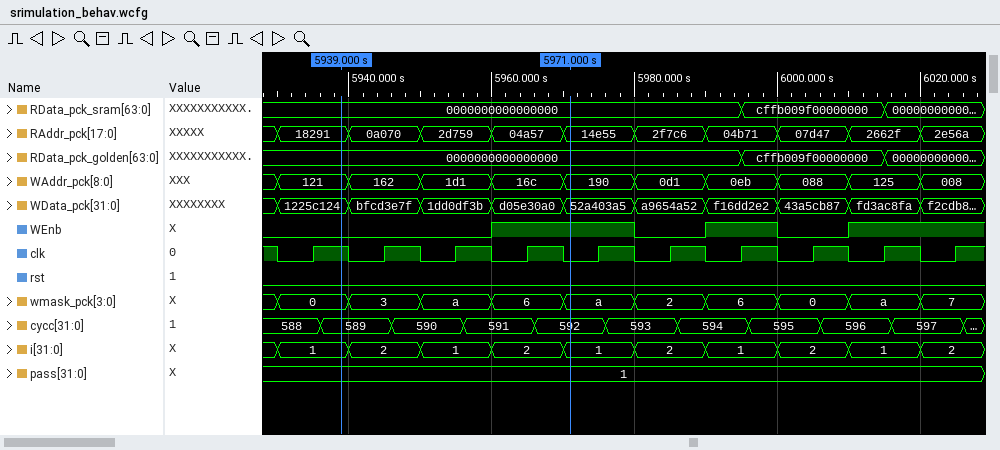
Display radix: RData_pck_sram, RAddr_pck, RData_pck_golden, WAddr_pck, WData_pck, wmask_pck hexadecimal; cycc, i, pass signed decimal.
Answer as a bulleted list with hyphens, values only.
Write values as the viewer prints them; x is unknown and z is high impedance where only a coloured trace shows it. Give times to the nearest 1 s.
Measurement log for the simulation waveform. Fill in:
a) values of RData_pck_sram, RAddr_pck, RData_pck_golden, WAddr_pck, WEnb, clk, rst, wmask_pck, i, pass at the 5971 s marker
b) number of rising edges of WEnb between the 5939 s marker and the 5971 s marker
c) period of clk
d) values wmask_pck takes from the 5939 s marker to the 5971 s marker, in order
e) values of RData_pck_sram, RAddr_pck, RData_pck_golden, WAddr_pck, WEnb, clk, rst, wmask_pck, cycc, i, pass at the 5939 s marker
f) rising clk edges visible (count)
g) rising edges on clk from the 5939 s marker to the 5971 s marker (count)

- RData_pck_sram=0000000000000000, RAddr_pck=14e55, RData_pck_golden=0000000000000000, WAddr_pck=190, WEnb=1, clk=0, rst=0, wmask_pck=a, i=1, pass=1
- 1
- 10 s
- 0, 3, a, 6, a
- RData_pck_sram=0000000000000000, RAddr_pck=18291, RData_pck_golden=0000000000000000, WAddr_pck=121, WEnb=0, clk=1, rst=0, wmask_pck=0, cycc=589, i=1, pass=1
- 10
- 3
